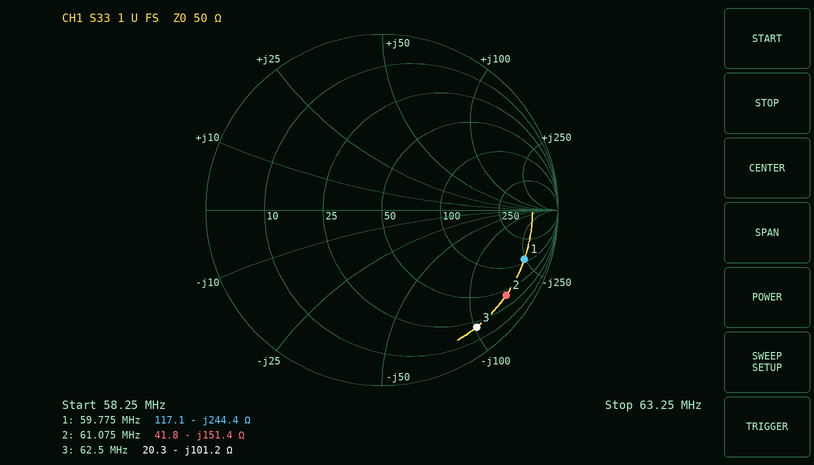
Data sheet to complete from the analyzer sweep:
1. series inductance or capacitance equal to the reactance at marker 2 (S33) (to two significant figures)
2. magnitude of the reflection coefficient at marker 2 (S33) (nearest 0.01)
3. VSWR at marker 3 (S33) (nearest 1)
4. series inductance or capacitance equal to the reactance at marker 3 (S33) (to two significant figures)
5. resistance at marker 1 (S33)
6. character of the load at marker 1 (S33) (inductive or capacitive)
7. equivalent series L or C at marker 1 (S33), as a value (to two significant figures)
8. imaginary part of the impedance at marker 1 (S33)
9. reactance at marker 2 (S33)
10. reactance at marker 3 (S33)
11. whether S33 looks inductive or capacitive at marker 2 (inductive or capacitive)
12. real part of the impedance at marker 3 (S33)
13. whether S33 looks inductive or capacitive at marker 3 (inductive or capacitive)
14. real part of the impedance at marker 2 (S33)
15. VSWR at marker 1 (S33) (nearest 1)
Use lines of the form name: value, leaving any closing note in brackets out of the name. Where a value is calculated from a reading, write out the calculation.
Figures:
series inductance or capacitance equal to the reactance at marker 2 (S33): C = 1/(2π × 61.075 MHz × 151.4 Ω) ≈ 17 pF
magnitude of the reflection coefficient at marker 2 (S33): 0.86
VSWR at marker 3 (S33): 13
series inductance or capacitance equal to the reactance at marker 3 (S33): C = 1/(2π × 62.5 MHz × 101.2 Ω) ≈ 25 pF
resistance at marker 1: 117.1 Ω
character of the load at marker 1 (S33): capacitive
equivalent series L or C at marker 1 (S33), as a value: C = 1/(2π × 59.775 MHz × 244.4 Ω) ≈ 11 pF
imaginary part of the impedance at marker 1: -244.4 Ω
reactance at marker 2: -151.4 Ω
reactance at marker 3: -101.2 Ω
whether S33 looks inductive or capacitive at marker 2: capacitive
real part of the impedance at marker 3: 20.3 Ω
whether S33 looks inductive or capacitive at marker 3: capacitive
real part of the impedance at marker 2: 41.8 Ω
VSWR at marker 1 (S33): 13
